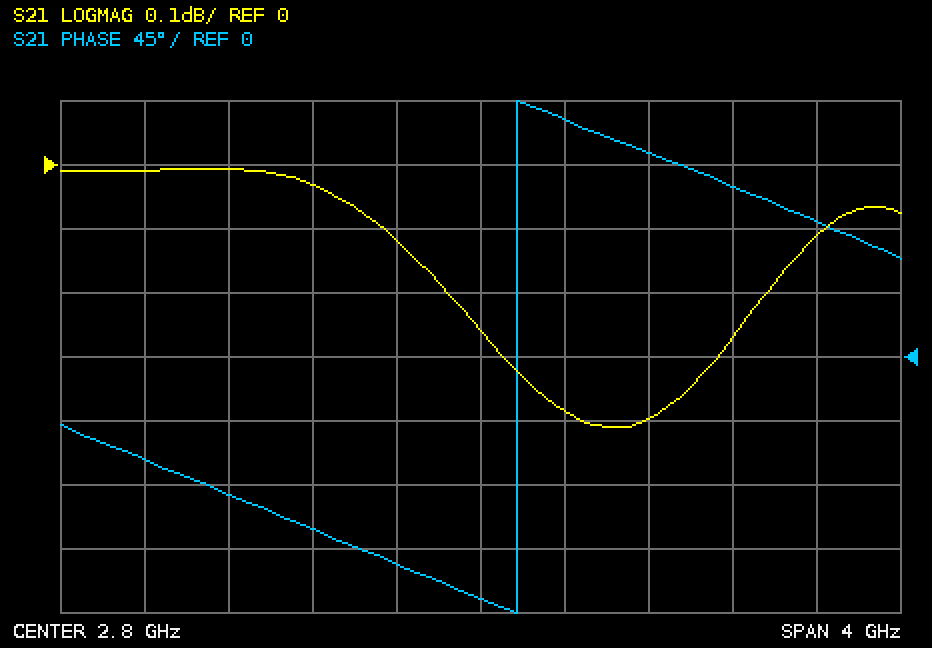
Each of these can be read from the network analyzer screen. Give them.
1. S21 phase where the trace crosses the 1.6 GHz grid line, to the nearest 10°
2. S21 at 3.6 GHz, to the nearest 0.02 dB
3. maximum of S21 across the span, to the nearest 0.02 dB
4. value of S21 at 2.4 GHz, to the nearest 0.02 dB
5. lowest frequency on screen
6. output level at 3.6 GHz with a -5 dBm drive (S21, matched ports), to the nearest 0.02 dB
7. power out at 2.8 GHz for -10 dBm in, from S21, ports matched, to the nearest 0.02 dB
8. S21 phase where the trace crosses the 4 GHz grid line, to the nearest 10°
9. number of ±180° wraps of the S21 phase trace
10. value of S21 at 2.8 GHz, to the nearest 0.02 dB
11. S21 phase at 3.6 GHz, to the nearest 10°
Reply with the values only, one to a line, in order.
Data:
-100°
-0.40 dB
0.00 dB
-0.12 dB
800 MHz
-5.40 dBm
-10.26 dBm
120°
1
-0.26 dB
140°
